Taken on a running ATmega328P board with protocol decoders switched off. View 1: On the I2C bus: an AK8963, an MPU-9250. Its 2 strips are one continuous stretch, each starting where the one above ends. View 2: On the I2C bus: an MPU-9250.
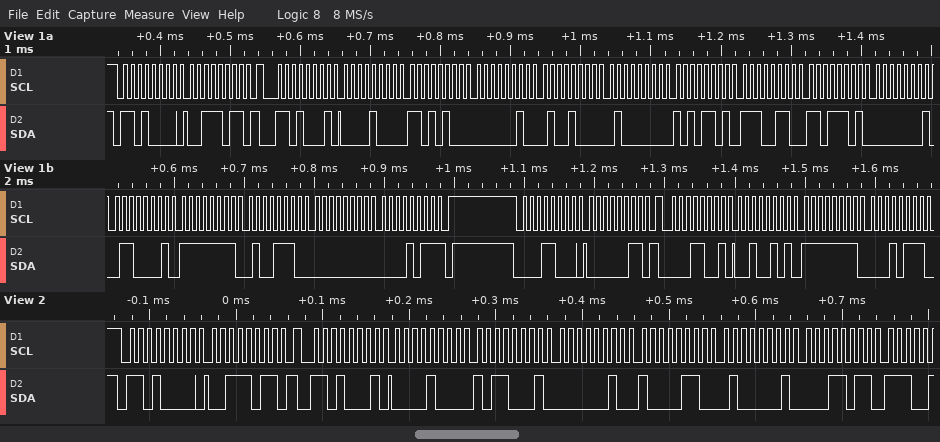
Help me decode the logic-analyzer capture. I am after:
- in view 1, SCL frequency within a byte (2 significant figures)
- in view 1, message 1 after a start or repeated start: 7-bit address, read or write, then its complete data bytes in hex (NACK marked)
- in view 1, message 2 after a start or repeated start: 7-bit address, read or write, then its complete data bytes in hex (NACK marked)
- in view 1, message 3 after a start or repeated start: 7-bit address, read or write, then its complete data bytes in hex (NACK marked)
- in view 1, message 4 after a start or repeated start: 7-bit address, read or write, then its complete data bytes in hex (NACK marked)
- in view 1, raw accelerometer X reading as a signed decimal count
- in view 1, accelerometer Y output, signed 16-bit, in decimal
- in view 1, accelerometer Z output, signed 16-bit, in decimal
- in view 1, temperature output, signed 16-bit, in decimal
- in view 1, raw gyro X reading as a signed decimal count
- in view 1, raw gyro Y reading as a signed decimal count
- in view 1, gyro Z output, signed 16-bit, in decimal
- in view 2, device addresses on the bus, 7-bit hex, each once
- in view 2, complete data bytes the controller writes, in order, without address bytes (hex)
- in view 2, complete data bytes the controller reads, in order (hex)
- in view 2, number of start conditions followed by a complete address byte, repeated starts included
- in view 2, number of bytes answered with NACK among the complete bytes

100 kHz
0x68 write: 3B
0x68 read: 08 D4 02 48 40 AD E6 DD 01 61 FF 4E 00 0B NACK
0x0C write: 03
0x0C read: 25 FF 17
2260
584
16557
-6435
353
-178
11
0x68
3B
08 B1 02 86 41 1B
2
0
